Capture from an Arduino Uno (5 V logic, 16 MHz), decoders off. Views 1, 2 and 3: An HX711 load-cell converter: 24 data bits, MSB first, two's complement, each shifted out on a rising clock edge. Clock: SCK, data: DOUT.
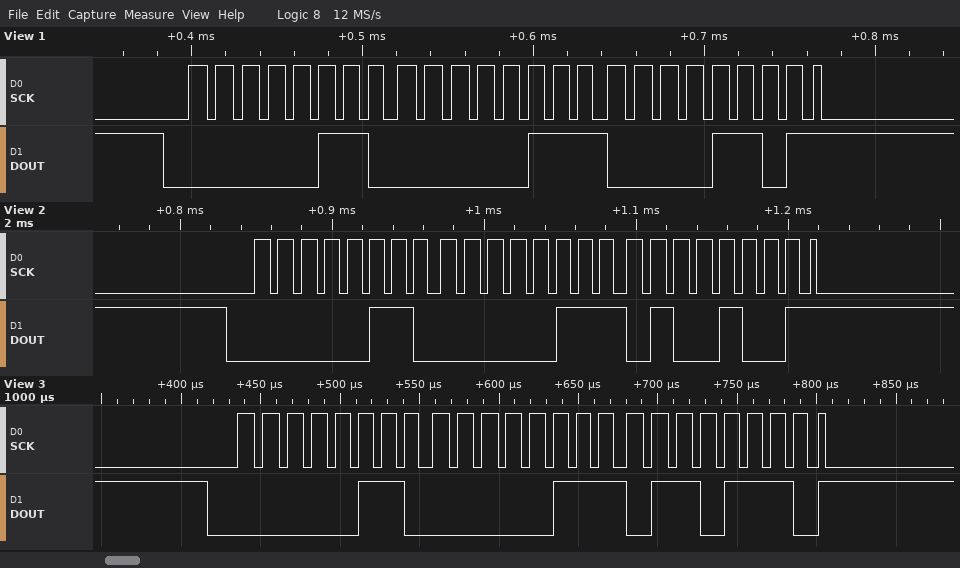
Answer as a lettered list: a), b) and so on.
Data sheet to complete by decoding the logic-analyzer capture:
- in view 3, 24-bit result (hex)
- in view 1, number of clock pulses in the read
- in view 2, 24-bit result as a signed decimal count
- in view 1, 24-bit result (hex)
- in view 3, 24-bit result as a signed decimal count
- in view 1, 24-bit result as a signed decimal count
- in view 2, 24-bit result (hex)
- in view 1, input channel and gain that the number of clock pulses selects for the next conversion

a) 0x06076E
b) 25
c) 395081
d) 0x06070D
e) 395118
f) 395021
g) 0x060749
h) channel A, gain 128
